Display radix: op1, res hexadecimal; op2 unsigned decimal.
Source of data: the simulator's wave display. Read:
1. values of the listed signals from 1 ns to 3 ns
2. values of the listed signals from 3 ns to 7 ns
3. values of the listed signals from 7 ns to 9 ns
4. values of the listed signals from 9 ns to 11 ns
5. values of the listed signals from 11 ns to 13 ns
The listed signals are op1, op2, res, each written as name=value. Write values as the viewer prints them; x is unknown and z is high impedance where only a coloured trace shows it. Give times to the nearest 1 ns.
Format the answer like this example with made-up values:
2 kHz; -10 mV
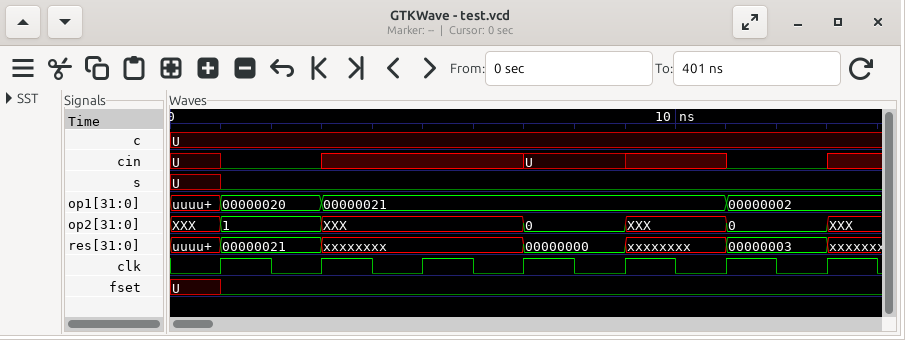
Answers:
op1=00000020, op2=1, res=00000021; op1=00000021, op2=XXX, res=xxxxxxxx; op1=00000021, op2=0, res=00000000; op1=00000021, op2=XXX, res=xxxxxxxx; op1=00000002, op2=0, res=00000003
